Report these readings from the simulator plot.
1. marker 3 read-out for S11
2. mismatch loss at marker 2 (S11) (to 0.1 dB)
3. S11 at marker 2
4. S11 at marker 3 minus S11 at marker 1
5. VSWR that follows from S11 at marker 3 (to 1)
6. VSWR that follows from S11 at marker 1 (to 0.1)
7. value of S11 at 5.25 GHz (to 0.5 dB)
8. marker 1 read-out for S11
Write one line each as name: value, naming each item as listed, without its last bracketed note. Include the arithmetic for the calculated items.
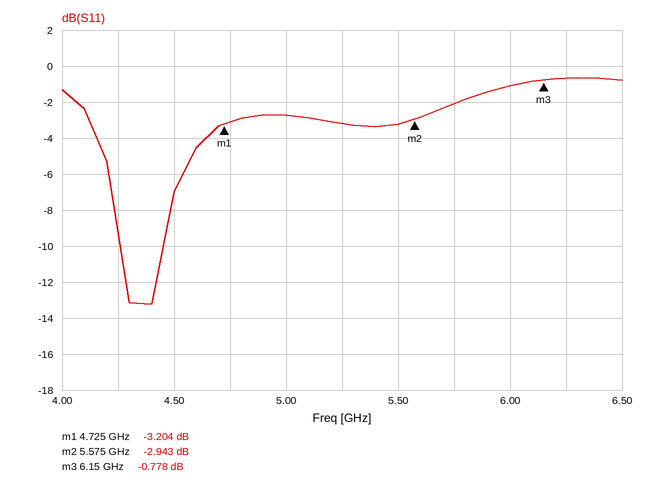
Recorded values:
marker 3 read-out for S11: -0.778 dB
mismatch loss at marker 2 (S11): −10 log10(1 − 10^(-2.943/10)) ≈ 3.1 dB
S11 at marker 2: -2.943 dB
S11 at marker 3 minus S11 at marker 1: -0.778 − (-3.204) = 2.426 dB
VSWR that follows from S11 at marker 3: (1 + 0.9143)/(1 − 0.9143) ≈ 22
VSWR that follows from S11 at marker 1: (1 + 0.6915)/(1 − 0.6915) ≈ 5.5
value of S11 at 5.25 GHz: -3.0 dB
marker 1 read-out for S11: -3.204 dB
